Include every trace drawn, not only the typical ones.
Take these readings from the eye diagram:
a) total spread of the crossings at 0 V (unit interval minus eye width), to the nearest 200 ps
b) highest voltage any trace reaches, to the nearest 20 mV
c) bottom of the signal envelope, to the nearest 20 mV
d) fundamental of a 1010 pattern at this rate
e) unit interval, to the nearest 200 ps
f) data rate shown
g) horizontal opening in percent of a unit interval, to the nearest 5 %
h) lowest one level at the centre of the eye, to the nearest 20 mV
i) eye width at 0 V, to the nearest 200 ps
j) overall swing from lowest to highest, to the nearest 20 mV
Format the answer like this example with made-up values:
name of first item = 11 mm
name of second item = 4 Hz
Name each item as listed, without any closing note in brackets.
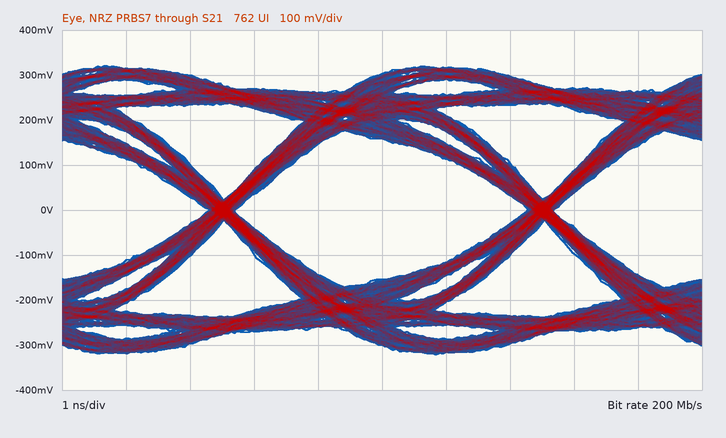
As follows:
total spread of the crossings at 0 V (unit interval minus eye width), to the nearest 200 ps = 400 ps
highest voltage any trace reaches, to the nearest 20 mV = 320 mV
bottom of the signal envelope, to the nearest 20 mV = -320 mV
fundamental of a 1010 pattern at this rate = 100 MHz
unit interval, to the nearest 200 ps = 5.0 ns
data rate shown = 200 Mb/s
horizontal opening in percent of a unit interval, to the nearest 5 % = 90 %
lowest one level at the centre of the eye, to the nearest 20 mV = 160 mV
eye width at 0 V, to the nearest 200 ps = 4.6 ns
overall swing from lowest to highest, to the nearest 20 mV = 640 mV
